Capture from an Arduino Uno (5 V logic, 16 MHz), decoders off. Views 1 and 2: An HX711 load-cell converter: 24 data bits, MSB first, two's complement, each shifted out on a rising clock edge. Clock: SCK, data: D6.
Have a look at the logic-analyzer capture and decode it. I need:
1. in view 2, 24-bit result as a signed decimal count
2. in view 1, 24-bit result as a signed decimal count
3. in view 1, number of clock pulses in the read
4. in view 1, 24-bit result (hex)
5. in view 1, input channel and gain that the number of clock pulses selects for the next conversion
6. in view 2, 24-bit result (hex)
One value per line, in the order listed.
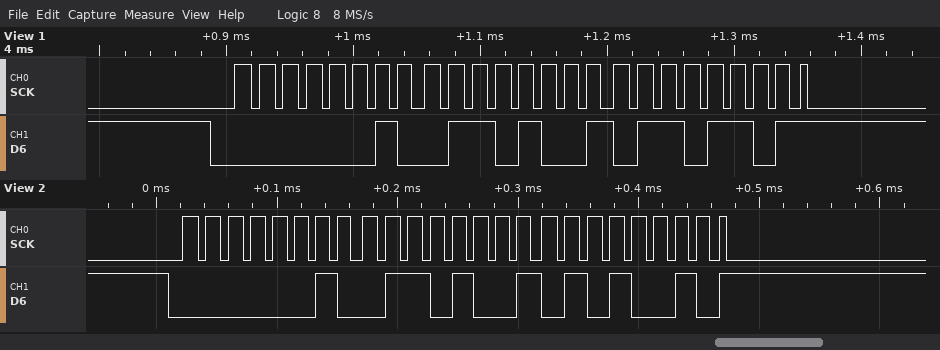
158034
158061
25
0x02696D
channel A, gain 128
0x026952
